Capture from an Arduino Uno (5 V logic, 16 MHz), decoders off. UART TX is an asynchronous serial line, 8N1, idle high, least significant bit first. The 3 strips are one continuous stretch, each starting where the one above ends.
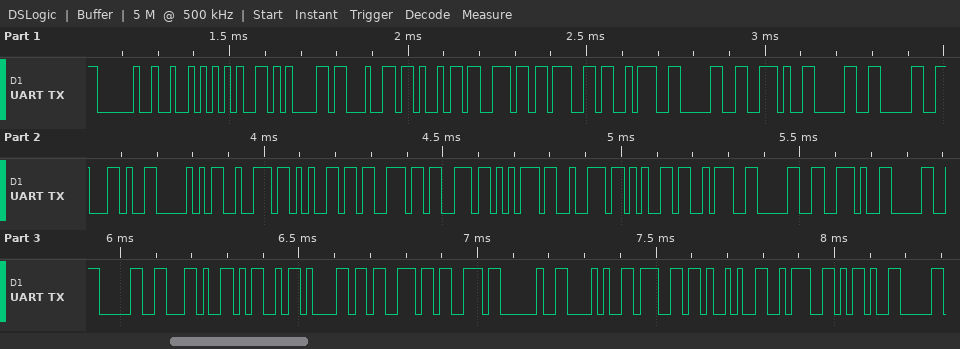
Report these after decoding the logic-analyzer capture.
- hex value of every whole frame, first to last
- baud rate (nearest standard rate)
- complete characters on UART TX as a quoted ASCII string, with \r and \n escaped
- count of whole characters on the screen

20 52 65 61 64 69 6E 67 3A 30 2E 30 30 2C 50 72 65 73 73 75 72 65 3A 30 2E 30 30 2C 4D 61 73 73 20 28 67 29 3A 2D
57600 baud
" Reading:0.00,Pressure:0.00,Mass (g):-"
38
